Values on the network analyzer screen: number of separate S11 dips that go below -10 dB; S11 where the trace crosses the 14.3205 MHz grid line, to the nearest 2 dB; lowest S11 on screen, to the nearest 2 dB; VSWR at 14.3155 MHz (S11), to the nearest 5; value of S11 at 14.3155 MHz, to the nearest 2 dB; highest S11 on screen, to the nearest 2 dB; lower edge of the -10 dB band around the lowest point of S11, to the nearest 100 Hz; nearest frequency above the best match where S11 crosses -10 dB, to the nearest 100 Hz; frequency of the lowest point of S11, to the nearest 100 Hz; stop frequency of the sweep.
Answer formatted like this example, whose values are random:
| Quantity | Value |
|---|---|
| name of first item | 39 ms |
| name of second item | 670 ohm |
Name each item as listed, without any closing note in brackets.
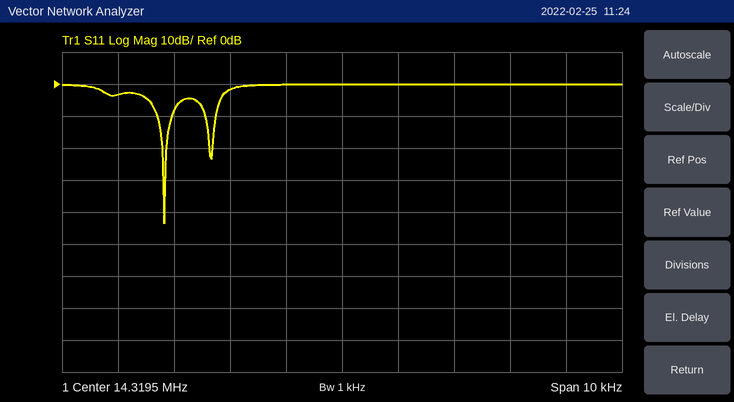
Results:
| Quantity | Value |
|---|---|
| number of separate S11 dips that go below -10 dB | 2 |
| S11 where the trace crosses the 14.3205 MHz grid line, to the nearest 2 dB | 0 dB |
| lowest S11 on screen, to the nearest 2 dB | -44 dB |
| VSWR at 14.3155 MHz (S11), to the nearest 5 | 5 |
| value of S11 at 14.3155 MHz, to the nearest 2 dB | -4 dB |
| highest S11 on screen, to the nearest 2 dB | 0 dB |
| lower edge of the -10 dB band around the lowest point of S11, to the nearest 100 Hz | 14.3162 MHz |
| nearest frequency above the best match where S11 crosses -10 dB, to the nearest 100 Hz | 14.3165 MHz |
| frequency of the lowest point of S11, to the nearest 100 Hz | 14.3163 MHz |
| stop frequency of the sweep | 14.3245 MHz |
